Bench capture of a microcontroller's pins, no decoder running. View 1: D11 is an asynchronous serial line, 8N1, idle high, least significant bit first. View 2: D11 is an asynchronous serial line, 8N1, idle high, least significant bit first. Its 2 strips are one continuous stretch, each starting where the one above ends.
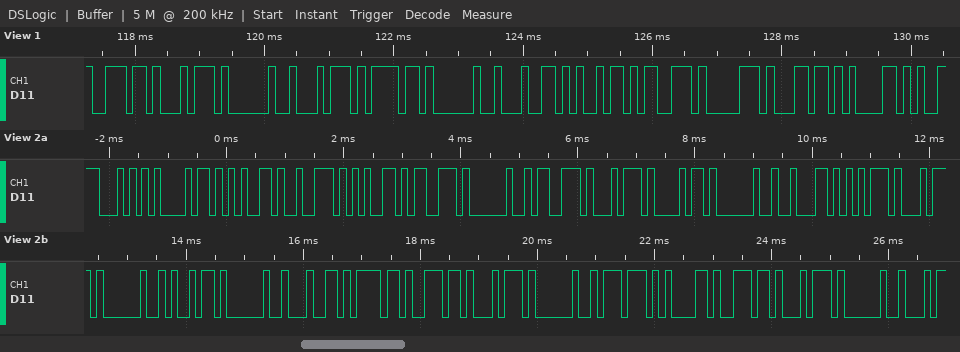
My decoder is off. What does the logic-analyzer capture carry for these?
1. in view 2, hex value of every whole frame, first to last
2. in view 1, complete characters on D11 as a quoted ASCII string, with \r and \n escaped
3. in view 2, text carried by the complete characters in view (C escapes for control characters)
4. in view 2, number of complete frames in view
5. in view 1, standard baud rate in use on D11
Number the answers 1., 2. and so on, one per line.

1. 54 68 65 72 65 73 20 73 74 68 20 62 75 74 20 69 20 64 6F 6E 74 20 77 61 6E 74 20
2. "nt to displa"
3. "Theres sth but i dont want "
4. 27
5. 9600 baud
